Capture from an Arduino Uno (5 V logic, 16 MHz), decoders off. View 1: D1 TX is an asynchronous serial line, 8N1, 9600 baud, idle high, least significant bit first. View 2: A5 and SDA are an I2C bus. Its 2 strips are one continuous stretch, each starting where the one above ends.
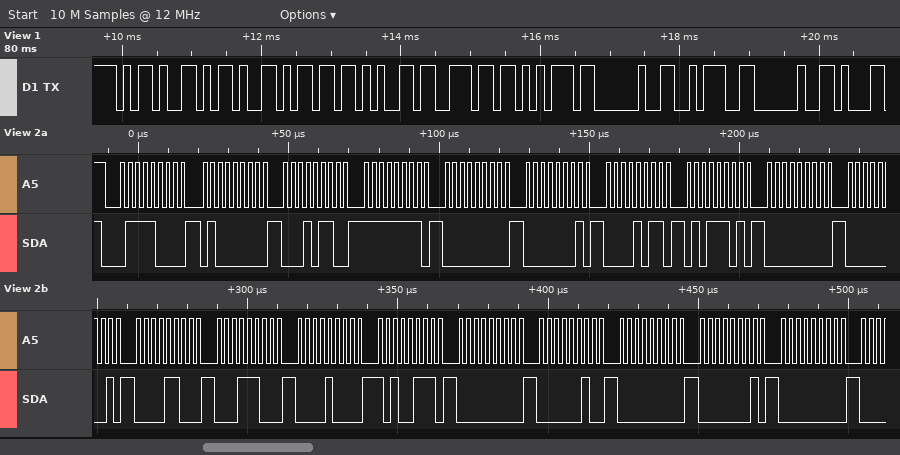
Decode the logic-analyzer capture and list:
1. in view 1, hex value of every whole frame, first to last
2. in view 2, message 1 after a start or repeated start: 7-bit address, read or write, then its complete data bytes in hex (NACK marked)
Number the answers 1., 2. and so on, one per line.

1. 2D 2D 6D 65 6E 75 20 3A 20
2. 0x3C write: 40 16 FF 00 01 0B 5D 00 01 0C 1C 08 A7 00 02 00 01 00
